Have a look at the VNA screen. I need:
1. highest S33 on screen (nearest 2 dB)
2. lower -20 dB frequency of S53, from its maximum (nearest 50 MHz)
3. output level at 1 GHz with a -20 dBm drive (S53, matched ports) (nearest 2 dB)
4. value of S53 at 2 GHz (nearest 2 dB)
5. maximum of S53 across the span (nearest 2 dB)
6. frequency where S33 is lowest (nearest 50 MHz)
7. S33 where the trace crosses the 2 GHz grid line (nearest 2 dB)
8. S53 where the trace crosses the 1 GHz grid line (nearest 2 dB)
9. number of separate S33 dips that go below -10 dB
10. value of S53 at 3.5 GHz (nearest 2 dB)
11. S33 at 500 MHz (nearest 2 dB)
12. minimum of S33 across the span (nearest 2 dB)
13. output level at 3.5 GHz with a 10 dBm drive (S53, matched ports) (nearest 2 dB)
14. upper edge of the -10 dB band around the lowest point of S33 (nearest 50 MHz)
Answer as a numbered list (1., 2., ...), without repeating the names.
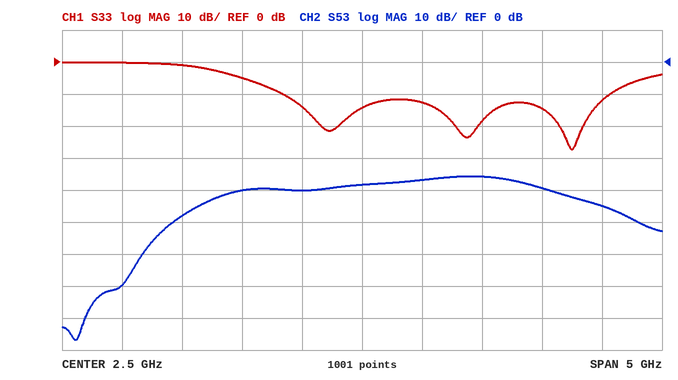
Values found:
1. 0 dB
2. 750 MHz
3. -68 dBm
4. -40 dB
5. -36 dB
6. 4.25 GHz
7. -14 dB
8. -48 dB
9. 3
10. -36 dB
11. 0 dB
12. -28 dB
13. -26 dBm
14. 4.55 GHz
